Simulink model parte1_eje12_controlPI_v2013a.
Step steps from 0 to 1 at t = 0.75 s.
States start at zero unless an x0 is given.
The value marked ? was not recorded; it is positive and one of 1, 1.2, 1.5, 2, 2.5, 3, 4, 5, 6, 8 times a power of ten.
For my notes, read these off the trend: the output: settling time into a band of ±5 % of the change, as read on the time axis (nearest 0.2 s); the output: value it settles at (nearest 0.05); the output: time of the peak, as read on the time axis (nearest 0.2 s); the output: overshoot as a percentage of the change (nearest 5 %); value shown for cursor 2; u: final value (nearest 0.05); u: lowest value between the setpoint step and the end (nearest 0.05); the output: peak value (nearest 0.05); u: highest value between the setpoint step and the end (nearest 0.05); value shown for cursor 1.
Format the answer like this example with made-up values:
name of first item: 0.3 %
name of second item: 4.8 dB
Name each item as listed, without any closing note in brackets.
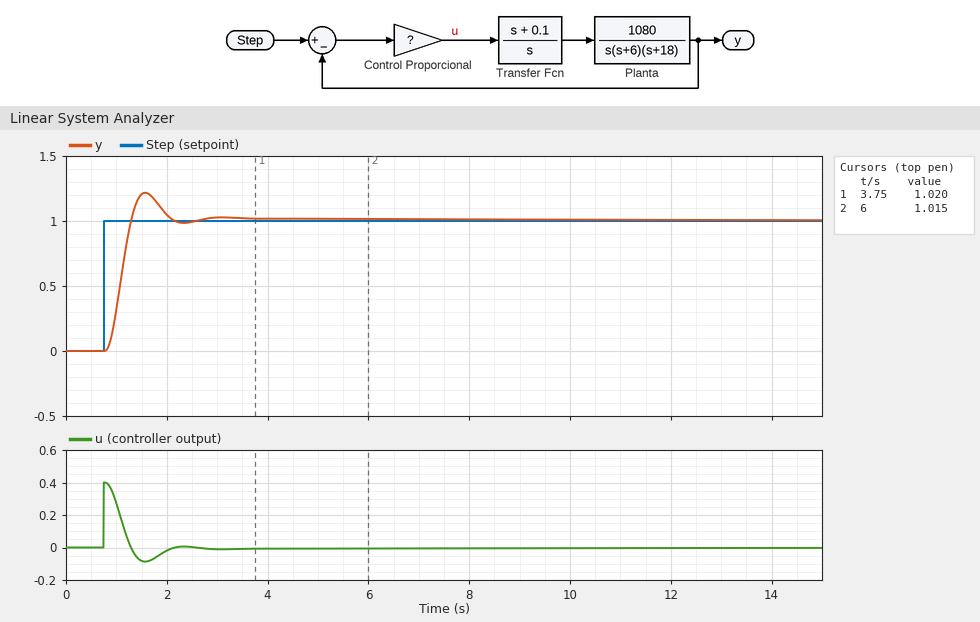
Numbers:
the output: settling time into a band of ±5 % of the change, as read on the time axis: 2.0 s
the output: value it settles at: 1.00
the output: time of the peak, as read on the time axis: 1.6 s
the output: overshoot as a percentage of the change: 20 %
value shown for cursor 2: 1.015
u: final value: 0.00
u: lowest value between the setpoint step and the end: -0.10
the output: peak value: 1.20
u: highest value between the setpoint step and the end: 0.40
value shown for cursor 1: 1.020
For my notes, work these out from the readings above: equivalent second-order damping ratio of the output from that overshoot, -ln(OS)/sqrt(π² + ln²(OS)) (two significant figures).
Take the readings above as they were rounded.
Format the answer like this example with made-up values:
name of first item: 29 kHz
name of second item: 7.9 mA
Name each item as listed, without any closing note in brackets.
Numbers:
equivalent second-order damping ratio of the output from that overshoot, -ln(OS)/sqrt(π² + ln²(OS)): 0.46
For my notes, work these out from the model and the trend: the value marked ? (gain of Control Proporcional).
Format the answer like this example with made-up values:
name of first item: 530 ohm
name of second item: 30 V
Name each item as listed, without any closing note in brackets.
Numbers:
the value marked ?: 0.4
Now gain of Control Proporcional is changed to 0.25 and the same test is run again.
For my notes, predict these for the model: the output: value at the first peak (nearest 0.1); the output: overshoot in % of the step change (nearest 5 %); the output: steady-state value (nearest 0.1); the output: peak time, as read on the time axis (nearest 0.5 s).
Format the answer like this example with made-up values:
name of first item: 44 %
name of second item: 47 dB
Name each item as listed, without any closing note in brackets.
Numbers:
the output: value at the first peak: 1.1
the output: overshoot in % of the step change: 10 %
the output: steady-state value: 1.0
the output: peak time, as read on the time axis: 2.0 s
